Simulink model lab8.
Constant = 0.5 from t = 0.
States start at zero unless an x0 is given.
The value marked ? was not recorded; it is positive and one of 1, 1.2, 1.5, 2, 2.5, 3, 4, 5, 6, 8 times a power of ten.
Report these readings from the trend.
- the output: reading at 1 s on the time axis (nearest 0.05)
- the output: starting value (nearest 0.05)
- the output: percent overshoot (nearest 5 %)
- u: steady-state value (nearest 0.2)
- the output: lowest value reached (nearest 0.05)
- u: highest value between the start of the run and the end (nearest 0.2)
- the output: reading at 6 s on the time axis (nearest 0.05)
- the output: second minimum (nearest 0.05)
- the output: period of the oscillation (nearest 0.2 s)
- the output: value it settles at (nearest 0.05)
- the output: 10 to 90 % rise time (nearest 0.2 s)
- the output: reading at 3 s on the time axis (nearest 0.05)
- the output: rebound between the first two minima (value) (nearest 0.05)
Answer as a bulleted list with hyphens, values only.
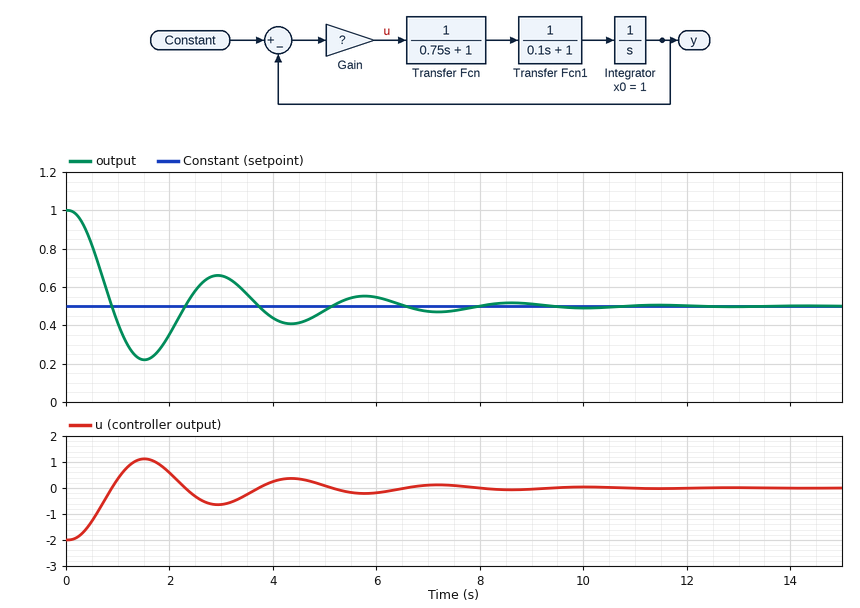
- 0.40
- 1.00
- 55 %
- 0.0
- 0.20
- 1.2
- 0.55
- 0.40
- 2.8 s
- 0.50
- 0.6 s
- 0.65
- 0.65
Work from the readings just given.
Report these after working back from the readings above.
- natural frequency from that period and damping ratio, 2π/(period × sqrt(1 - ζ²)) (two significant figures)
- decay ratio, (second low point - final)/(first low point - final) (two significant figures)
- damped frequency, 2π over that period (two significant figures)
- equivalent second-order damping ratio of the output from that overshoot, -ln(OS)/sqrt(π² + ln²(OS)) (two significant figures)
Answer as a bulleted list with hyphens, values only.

- 2.3 rad/s
- 0.33
- 2.2 rad/s
- 0.19
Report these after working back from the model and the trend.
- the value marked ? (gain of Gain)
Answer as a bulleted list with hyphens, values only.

- 4
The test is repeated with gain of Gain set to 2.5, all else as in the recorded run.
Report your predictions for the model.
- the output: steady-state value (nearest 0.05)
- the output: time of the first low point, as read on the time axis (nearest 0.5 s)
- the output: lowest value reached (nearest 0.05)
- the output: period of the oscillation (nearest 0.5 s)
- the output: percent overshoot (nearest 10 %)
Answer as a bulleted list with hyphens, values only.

- 0.50
- 2.0 s
- 0.30
- 3.5 s
- 40 %
